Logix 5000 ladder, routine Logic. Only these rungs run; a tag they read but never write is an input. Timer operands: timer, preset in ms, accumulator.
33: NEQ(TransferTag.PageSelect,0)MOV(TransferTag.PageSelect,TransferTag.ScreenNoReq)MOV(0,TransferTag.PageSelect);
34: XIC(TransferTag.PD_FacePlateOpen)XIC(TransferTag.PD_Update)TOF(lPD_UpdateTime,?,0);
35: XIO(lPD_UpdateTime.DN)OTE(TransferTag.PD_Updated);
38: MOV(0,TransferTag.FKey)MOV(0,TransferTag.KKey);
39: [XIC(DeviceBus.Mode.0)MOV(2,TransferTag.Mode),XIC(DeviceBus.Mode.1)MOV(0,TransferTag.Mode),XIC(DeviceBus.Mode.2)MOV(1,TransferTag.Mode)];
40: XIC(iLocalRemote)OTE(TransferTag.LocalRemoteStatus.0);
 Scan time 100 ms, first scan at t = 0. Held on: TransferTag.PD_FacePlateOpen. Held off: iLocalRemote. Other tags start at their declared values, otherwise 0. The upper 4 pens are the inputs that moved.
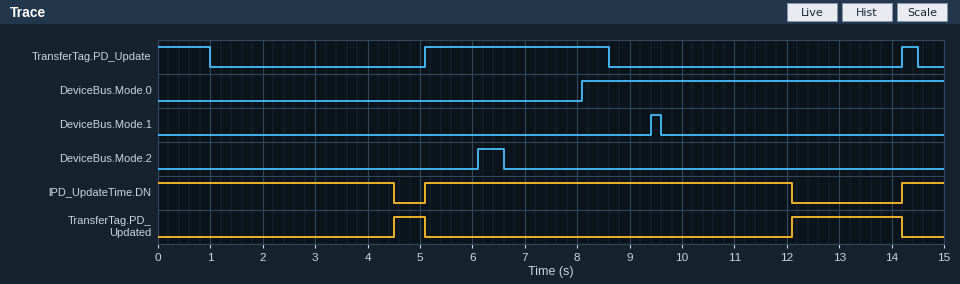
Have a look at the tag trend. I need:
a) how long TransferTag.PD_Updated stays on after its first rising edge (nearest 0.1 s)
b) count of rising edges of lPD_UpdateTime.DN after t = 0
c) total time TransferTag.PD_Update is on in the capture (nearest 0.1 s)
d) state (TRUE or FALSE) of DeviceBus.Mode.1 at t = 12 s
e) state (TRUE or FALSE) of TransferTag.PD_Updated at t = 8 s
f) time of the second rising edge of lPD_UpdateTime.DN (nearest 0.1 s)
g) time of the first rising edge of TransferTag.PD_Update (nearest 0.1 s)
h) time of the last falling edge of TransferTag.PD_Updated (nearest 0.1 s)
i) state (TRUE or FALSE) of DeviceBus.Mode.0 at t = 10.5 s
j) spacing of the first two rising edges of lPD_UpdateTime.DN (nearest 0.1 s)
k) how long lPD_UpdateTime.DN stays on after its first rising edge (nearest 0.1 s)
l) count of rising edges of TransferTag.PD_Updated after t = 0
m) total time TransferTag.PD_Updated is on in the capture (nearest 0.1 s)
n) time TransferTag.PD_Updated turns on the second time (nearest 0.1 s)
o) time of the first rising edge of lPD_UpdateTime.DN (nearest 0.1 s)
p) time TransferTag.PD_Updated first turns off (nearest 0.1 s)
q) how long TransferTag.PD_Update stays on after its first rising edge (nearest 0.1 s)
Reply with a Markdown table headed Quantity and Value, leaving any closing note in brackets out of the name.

| Quantity | Value |
|---|---|
| how long TransferTag.PD_Updated stays on after its first rising edge | 0.6 s |
| count of rising edges of lPD_UpdateTime.DN after t = 0 | 2 |
| total time TransferTag.PD_Update is on in the capture | 4.8 s |
| state (TRUE or FALSE) of DeviceBus.Mode.1 at t = 12 s | FALSE |
| state (TRUE or FALSE) of TransferTag.PD_Updated at t = 8 s | FALSE |
| time of the second rising edge of lPD_UpdateTime.DN | 14.2 s |
| time of the first rising edge of TransferTag.PD_Update | 5.1 s |
| time of the last falling edge of TransferTag.PD_Updated | 14.2 s |
| state (TRUE or FALSE) of DeviceBus.Mode.0 at t = 10.5 s | TRUE |
| spacing of the first two rising edges of lPD_UpdateTime.DN | 9.1 s |
| how long lPD_UpdateTime.DN stays on after its first rising edge | 7.0 s |
| count of rising edges of TransferTag.PD_Updated after t = 0 | 2 |
| total time TransferTag.PD_Updated is on in the capture | 2.7 s |
| time TransferTag.PD_Updated turns on the second time | 12.1 s |
| time of the first rising edge of lPD_UpdateTime.DN | 5.1 s |
| time TransferTag.PD_Updated first turns off | 5.1 s |
| how long TransferTag.PD_Update stays on after its first rising edge | 3.5 s |
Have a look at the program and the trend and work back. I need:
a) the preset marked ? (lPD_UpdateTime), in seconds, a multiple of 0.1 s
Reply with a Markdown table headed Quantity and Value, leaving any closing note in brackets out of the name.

| Quantity | Value |
|---|---|
| the preset marked ? (lPD_UpdateTime), in seconds, a multiple of 0.1 s | 3.5 s |
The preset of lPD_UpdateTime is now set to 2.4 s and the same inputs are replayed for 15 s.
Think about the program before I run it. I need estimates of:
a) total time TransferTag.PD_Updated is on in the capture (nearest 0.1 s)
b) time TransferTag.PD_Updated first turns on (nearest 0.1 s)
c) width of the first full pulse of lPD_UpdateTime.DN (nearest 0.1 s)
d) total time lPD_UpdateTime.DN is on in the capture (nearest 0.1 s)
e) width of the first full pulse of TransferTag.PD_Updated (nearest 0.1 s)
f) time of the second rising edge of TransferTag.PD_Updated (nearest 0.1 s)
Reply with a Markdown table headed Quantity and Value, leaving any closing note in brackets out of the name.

| Quantity | Value |
|---|---|
| total time TransferTag.PD_Updated is on in the capture | 4.9 s |
| time TransferTag.PD_Updated first turns on | 3.4 s |
| width of the first full pulse of lPD_UpdateTime.DN | 5.9 s |
| total time lPD_UpdateTime.DN is on in the capture | 10.1 s |
| width of the first full pulse of TransferTag.PD_Updated | 1.7 s |
| time of the second rising edge of TransferTag.PD_Updated | 11.0 s |
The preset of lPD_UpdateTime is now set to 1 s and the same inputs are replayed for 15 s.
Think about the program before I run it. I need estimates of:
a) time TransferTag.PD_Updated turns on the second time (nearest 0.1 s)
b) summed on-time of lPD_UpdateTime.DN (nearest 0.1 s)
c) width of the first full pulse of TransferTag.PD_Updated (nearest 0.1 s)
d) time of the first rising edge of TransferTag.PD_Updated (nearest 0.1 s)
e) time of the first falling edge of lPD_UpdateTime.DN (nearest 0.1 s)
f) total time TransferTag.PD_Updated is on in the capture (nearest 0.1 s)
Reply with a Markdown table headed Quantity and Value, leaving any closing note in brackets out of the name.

| Quantity | Value |
|---|---|
| time TransferTag.PD_Updated turns on the second time | 9.6 s |
| summed on-time of lPD_UpdateTime.DN | 7.3 s |
| width of the first full pulse of TransferTag.PD_Updated | 3.1 s |
| time of the first rising edge of TransferTag.PD_Updated | 2.0 s |
| time of the first falling edge of lPD_UpdateTime.DN | 2.0 s |
| total time TransferTag.PD_Updated is on in the capture | 7.7 s |
